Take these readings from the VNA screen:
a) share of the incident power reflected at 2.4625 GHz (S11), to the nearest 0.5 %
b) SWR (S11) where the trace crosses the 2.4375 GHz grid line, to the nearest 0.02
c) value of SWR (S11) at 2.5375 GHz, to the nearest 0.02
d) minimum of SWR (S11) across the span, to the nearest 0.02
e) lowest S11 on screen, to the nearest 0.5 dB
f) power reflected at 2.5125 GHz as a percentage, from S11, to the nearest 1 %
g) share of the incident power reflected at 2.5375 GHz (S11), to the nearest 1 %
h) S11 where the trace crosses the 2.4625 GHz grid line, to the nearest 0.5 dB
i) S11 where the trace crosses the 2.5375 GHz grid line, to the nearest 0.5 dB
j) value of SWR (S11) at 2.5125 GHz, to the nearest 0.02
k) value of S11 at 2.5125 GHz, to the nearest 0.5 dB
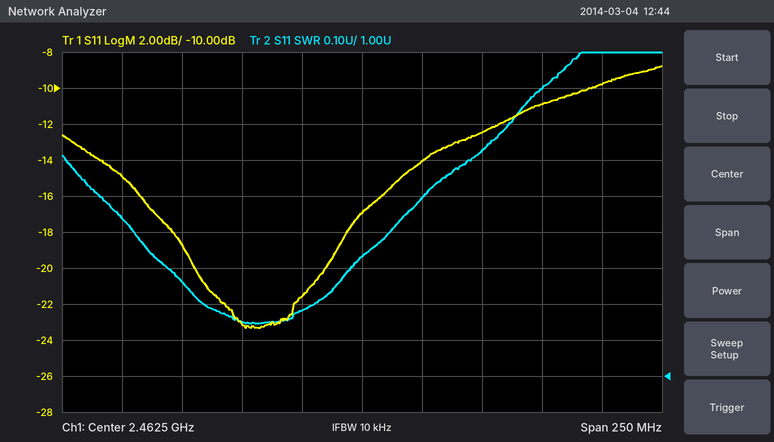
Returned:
2.0 %
1.18
1.80
1.14
-23.5 dB
6 %
8 %
-17.0 dB
-11.0 dB
1.62
-12.5 dB
